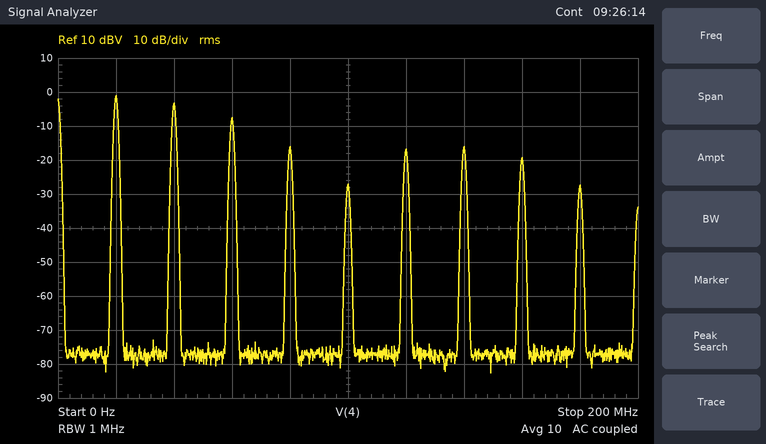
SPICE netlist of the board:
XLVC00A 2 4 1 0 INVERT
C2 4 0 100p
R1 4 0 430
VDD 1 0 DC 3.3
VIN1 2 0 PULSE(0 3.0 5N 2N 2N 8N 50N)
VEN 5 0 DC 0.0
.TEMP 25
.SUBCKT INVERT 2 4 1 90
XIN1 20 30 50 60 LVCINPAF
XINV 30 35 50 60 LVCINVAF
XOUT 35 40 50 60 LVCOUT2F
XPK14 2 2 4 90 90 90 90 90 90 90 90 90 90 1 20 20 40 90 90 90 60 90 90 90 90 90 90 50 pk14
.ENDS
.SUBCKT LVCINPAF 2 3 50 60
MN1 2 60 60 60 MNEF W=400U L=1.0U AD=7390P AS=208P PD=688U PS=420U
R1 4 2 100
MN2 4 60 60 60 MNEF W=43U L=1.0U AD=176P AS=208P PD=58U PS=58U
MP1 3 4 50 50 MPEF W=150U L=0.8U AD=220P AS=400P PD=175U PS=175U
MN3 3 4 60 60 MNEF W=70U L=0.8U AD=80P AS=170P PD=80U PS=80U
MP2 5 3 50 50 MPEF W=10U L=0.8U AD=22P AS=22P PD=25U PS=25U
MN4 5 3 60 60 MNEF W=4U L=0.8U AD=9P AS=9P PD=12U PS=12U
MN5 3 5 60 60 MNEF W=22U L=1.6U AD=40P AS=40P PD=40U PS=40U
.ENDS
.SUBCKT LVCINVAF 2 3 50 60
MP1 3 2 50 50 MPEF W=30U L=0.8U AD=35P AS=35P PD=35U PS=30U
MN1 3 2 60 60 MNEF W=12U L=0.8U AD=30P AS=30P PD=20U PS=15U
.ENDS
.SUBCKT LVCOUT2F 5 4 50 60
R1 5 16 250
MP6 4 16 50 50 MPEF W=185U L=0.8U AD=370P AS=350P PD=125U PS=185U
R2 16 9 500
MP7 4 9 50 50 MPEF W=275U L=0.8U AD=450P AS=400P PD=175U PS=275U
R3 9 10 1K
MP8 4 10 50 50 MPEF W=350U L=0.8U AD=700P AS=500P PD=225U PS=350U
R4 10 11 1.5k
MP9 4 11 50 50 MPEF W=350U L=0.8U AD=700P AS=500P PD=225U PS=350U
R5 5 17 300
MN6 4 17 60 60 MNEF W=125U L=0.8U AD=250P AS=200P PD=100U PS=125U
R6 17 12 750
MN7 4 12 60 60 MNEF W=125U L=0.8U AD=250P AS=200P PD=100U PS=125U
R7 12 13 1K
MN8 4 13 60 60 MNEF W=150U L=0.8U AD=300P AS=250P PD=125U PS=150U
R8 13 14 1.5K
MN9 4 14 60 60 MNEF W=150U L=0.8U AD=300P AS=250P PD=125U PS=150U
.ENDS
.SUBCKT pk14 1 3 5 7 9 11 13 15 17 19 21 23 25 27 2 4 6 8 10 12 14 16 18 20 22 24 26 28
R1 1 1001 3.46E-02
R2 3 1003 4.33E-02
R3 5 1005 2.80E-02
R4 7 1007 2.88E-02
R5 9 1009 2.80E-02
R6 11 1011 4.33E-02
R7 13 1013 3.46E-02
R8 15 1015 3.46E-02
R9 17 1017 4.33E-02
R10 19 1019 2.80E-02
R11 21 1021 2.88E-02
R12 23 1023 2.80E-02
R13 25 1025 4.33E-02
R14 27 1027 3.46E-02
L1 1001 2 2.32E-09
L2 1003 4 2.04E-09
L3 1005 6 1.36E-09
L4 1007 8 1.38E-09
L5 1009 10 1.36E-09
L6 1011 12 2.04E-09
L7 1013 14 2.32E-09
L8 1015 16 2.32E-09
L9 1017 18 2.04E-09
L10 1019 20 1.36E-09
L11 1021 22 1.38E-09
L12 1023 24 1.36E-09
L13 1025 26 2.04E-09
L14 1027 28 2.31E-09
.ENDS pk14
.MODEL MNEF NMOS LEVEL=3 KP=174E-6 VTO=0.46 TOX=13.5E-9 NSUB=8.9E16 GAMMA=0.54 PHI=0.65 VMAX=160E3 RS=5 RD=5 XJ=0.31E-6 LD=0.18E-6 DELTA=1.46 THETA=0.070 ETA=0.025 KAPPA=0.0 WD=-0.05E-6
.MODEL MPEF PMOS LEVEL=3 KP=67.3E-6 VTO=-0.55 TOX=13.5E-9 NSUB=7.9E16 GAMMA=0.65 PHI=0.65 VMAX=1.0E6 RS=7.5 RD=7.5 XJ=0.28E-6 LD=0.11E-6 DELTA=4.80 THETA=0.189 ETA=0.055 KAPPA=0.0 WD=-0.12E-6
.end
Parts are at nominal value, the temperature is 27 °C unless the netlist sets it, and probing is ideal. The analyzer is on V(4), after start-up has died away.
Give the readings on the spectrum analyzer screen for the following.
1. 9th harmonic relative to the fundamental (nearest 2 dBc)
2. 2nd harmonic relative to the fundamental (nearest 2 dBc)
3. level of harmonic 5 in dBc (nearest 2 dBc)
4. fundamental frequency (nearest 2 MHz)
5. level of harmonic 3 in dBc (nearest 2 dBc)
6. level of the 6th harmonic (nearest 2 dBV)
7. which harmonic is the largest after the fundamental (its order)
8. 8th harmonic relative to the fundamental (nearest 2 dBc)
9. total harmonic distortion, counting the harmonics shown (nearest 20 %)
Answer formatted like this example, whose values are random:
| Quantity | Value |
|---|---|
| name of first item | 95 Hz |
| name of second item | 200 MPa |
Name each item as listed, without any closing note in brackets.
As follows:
| Quantity | Value |
|---|---|
| 9th harmonic relative to the fundamental | -26 dBc |
| 2nd harmonic relative to the fundamental | -2 dBc |
| level of harmonic 5 in dBc | -26 dBc |
| fundamental frequency | 20 MHz |
| level of harmonic 3 in dBc | -6 dBc |
| level of the 6th harmonic | -16 dBV |
| which harmonic is the largest after the fundamental | 2 |
| 8th harmonic relative to the fundamental | -18 dBc |
| total harmonic distortion, counting the harmonics shown | 100 % |
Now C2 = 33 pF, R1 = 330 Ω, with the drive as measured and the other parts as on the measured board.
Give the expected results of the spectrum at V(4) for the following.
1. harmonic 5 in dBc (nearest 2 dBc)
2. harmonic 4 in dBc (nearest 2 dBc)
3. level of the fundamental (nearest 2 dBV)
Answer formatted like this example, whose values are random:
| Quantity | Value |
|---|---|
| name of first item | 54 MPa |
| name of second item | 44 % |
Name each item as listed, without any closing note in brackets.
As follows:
| Quantity | Value |
|---|---|
| harmonic 5 in dBc | -30 dBc |
| harmonic 4 in dBc | -14 dBc |
| level of the fundamental | -2 dBV |
